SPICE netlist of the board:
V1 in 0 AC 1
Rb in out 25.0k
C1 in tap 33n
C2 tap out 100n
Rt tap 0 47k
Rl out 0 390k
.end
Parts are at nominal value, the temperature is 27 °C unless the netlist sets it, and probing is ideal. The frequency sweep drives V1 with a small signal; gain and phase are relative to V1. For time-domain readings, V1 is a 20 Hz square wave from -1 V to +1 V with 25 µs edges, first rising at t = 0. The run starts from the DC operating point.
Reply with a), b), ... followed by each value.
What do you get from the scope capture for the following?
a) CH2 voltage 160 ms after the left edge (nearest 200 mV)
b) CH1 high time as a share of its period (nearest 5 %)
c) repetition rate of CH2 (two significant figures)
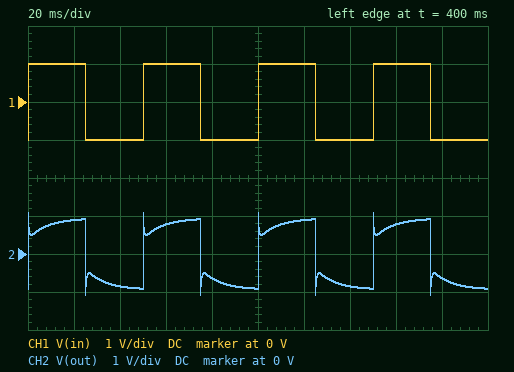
a) 800 mV
b) 50 %
c) 20 Hz
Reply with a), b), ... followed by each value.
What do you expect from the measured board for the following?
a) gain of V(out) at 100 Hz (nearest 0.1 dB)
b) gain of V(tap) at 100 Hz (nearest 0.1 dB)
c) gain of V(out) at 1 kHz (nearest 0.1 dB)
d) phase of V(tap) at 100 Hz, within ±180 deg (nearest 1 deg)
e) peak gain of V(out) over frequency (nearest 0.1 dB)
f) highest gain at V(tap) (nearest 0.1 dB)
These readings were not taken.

a) -3.3 dB
b) -2.6 dB
c) -0.3 dB
d) 16 deg
e) 0 dB
f) 0 dB
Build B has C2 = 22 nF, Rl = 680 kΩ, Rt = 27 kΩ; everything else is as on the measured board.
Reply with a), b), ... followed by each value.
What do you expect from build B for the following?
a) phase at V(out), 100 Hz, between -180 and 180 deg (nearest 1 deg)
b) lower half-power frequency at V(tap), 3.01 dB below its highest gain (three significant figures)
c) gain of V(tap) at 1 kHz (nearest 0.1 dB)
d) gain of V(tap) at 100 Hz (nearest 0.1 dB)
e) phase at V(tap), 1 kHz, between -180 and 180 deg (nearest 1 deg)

a) -8 deg
b) 138 Hz
c) -0.4 dB
d) -4.1 dB
e) 9 deg
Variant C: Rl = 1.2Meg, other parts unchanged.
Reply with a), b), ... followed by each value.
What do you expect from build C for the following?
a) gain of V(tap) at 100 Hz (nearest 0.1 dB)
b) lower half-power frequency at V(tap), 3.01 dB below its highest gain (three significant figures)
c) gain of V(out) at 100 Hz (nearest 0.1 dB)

a) -2.4 dB
b) 52.4 Hz
c) -3.0 dB
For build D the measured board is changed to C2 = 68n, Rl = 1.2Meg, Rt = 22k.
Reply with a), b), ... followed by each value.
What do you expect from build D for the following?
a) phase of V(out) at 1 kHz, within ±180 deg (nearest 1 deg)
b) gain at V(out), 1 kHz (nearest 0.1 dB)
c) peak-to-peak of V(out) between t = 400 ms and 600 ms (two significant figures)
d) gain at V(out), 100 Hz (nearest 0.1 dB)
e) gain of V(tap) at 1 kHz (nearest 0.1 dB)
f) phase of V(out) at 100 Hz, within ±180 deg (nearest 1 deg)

a) 11 deg
b) -0.7 dB
c) 2.0 V
d) -4.7 dB
e) -0.5 dB
f) -8 deg
